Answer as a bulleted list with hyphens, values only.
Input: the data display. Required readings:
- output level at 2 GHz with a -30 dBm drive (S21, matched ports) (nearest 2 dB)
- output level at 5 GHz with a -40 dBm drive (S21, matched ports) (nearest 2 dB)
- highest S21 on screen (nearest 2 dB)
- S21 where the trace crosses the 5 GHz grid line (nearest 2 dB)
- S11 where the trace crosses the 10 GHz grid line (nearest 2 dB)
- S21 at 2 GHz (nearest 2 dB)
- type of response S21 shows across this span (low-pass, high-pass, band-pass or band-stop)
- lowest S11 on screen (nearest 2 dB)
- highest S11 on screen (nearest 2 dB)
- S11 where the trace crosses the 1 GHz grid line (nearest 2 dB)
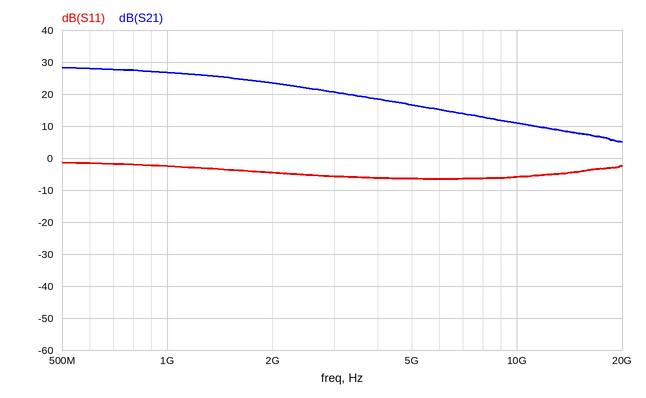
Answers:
- -6 dBm
- -24 dBm
- 28 dB
- 16 dB
- -6 dB
- 24 dB
- low-pass
- -6 dB
- -2 dB
- -2 dB
